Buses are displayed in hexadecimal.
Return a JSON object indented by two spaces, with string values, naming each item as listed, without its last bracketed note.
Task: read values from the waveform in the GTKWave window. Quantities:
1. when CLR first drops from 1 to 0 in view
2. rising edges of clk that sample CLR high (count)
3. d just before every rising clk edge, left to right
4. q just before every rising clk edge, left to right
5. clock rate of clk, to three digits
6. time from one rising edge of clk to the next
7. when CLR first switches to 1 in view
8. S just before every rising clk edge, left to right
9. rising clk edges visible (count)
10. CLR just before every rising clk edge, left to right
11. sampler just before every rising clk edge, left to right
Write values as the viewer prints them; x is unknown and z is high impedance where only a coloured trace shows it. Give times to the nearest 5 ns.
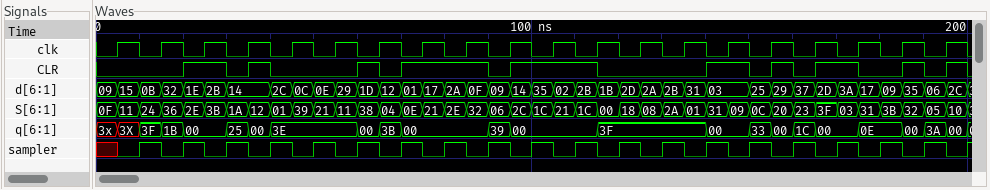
{
  "when CLR first drops from 1 to 0 in view": "30 ns",
  "rising edges of clk that sample CLR high": "8",
  "d just before every rising clk edge, left to right": "09, 0B, 1E, 14, 2C, 0E, 1D, 01, 2A, 09, 35, 2B, 2D, 2B, 03, 25, 37, 3A, 09, 06",
  "q just before every rising clk edge, left to right": "3x, 3F, 00, 25, 3E, 3E, 00, 00, 00, 39, 00, 00, 3F, 3F, 00, 33, 1C, 00, 0E, 3A",
  "clock rate of clk, to three digits": "100 MHz",
  "time from one rising edge of clk to the next": "10 ns",
  "when CLR first switches to 1 in view": "20 ns",
  "S just before every rising clk edge, left to right": "0F, 24, 2E, 1A, 01, 21, 38, 0E, 2E, 06, 1C, 1C, 18, 2A, 31, 0C, 23, 03, 3B, 05",
  "rising clk edges visible": "20",
  "CLR just before every rising clk edge, left to right": "0 0 1 0 0 0 1 1 1 0 1 1 0 0 1 0 0 1 0 0",
  "sampler just before every rising clk edge, left to right": "x 1 1 1 1 1 1 1 1 1 1 1 1 1 1 1 1 1 1 1"
}
